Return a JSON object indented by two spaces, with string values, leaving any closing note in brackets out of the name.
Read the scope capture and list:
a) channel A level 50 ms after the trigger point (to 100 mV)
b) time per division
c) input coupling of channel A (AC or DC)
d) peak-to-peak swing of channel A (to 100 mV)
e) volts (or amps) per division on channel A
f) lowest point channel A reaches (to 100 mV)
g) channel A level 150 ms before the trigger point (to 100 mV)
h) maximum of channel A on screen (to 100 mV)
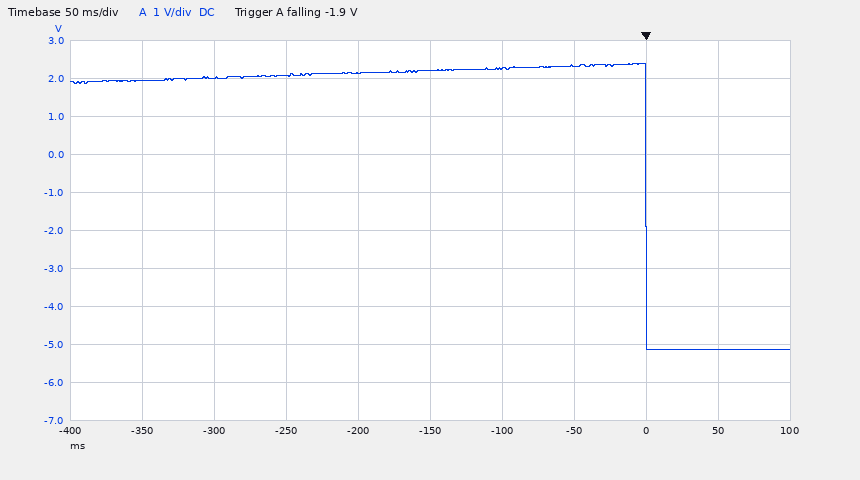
{
  "channel A level 50 ms after the trigger point": "-5.1 V",
  "time per division": "50 ms",
  "input coupling of channel A": "DC",
  "peak-to-peak swing of channel A": "7.5 V",
  "volts (or amps) per division on channel A": "1 V",
  "lowest point channel A reaches": "-5.1 V",
  "channel A level 150 ms before the trigger point": "2.2 V",
  "maximum of channel A on screen": "2.4 V"
}
